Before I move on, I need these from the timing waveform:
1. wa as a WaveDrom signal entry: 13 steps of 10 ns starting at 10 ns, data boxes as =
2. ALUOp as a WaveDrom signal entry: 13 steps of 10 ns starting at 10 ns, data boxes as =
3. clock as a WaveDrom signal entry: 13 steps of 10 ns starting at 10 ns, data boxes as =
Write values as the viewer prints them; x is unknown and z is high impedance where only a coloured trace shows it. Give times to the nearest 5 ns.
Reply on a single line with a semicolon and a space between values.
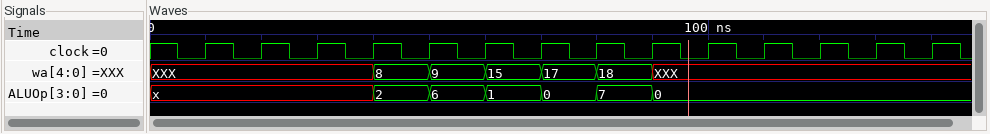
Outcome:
{name: 'wa', wave: 'x..=====x....', data: '8 9 15 17 18'}; {name: 'ALUOp', wave: 'x..======....', data: '2 6 1 0 7 0'}; {name: 'clock', wave: 'p............'}
